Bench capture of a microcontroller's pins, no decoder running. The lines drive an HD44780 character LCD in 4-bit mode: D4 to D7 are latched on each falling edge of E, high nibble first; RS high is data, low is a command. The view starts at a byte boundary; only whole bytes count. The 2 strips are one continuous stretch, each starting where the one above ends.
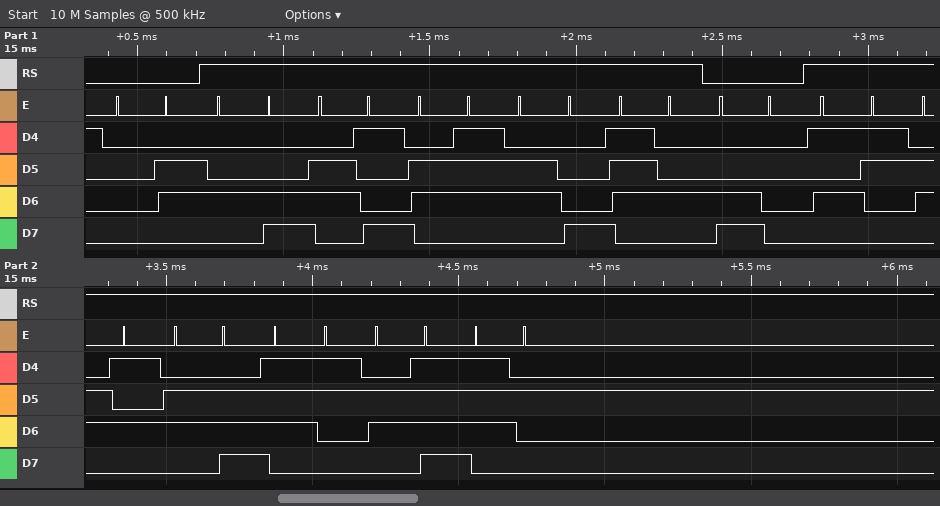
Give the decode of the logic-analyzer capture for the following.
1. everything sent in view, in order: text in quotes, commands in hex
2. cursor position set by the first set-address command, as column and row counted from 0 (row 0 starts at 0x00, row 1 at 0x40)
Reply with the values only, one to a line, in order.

0x06 "Light" 0xC0 "Sensor"
column 0, row 1
